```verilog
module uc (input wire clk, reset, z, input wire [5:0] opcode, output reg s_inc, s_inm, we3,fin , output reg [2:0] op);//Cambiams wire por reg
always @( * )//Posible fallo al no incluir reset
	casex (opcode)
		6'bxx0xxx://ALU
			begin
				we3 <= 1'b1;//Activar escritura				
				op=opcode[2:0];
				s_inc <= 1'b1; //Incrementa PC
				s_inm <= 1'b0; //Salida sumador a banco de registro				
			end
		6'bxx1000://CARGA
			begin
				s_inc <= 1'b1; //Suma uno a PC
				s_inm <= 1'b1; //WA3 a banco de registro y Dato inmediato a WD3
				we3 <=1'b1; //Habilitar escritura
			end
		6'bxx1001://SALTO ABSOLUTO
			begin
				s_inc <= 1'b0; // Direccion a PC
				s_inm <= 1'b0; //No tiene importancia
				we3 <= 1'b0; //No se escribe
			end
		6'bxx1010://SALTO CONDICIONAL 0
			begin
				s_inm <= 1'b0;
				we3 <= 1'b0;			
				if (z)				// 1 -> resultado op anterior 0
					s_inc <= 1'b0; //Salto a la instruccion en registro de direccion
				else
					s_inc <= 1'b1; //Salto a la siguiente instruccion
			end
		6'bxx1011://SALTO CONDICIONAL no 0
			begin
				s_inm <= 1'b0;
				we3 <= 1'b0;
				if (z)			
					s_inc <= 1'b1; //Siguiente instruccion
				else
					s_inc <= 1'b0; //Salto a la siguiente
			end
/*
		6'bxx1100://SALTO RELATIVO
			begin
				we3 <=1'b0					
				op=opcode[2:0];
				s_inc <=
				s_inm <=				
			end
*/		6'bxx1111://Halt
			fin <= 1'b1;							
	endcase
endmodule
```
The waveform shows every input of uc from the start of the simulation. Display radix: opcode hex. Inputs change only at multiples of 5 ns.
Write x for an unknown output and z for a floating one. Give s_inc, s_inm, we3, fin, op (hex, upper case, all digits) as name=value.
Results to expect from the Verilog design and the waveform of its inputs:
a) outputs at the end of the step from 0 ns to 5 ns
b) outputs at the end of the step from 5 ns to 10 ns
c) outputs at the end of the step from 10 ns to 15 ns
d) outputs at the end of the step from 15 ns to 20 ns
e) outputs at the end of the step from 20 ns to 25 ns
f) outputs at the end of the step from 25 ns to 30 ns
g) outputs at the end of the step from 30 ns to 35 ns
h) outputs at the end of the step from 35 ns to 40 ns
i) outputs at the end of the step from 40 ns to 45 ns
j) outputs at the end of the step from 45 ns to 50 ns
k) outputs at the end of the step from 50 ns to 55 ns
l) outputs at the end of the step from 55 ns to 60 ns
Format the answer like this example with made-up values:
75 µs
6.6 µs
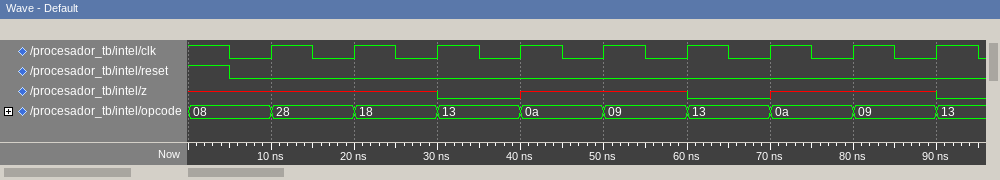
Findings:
s_inc=1, s_inm=1, we3=1, fin=x, op=x
s_inc=1, s_inm=1, we3=1, fin=x, op=x
s_inc=1, s_inm=1, we3=1, fin=x, op=x
s_inc=1, s_inm=1, we3=1, fin=x, op=x
s_inc=1, s_inm=1, we3=1, fin=x, op=x
s_inc=1, s_inm=1, we3=1, fin=x, op=x
s_inc=1, s_inm=0, we3=1, fin=x, op=3
s_inc=1, s_inm=0, we3=1, fin=x, op=3
s_inc=1, s_inm=0, we3=0, fin=x, op=3
s_inc=1, s_inm=0, we3=0, fin=x, op=3
s_inc=0, s_inm=0, we3=0, fin=x, op=3
s_inc=0, s_inm=0, we3=0, fin=x, op=3
